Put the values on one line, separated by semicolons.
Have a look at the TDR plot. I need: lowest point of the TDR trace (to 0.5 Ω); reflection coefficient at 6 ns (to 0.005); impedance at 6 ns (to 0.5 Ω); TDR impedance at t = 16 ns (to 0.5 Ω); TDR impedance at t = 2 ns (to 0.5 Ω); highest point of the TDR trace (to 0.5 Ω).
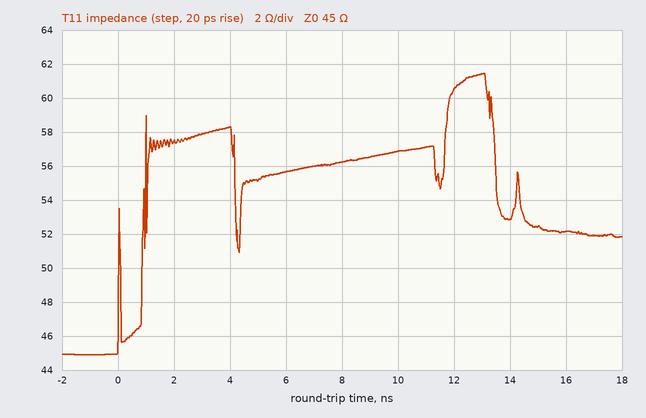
45.0 Ω; +0.105; 55.5 Ω; 52.0 Ω; 57.5 Ω; 61.5 Ω
